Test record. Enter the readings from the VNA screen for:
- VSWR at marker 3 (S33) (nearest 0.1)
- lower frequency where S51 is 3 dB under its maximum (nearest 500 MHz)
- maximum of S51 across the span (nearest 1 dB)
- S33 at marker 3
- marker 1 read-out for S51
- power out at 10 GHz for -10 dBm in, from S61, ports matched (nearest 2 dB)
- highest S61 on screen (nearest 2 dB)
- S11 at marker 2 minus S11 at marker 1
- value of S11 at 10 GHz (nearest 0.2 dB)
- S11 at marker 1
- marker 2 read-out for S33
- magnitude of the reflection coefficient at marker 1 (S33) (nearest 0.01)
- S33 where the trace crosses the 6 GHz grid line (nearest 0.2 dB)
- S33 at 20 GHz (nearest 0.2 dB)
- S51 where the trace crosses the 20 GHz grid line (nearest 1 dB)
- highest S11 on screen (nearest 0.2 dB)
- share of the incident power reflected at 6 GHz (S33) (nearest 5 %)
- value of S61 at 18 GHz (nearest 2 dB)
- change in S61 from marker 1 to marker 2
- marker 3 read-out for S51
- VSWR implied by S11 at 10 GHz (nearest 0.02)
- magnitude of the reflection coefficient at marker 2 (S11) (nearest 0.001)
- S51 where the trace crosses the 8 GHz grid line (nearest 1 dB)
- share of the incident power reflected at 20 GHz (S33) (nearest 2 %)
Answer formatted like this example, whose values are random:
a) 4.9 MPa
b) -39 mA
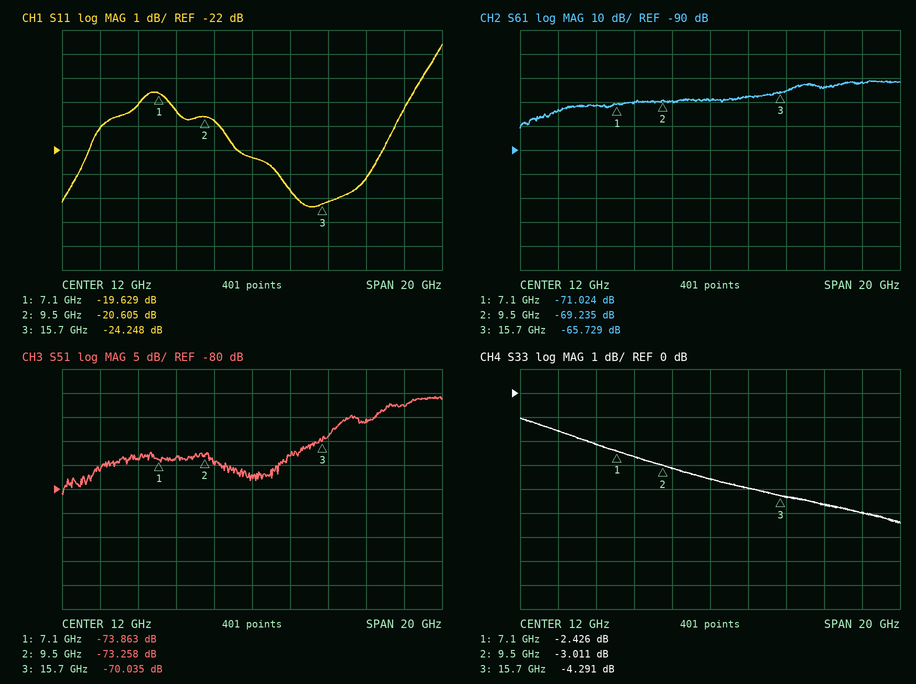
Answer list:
a) 4.1
b) 19.0 GHz
c) -61 dB
d) -4.291 dB
e) -73.863 dB
f) -80 dBm
g) -62 dB
h) -0.976 dB
i) -20.8 dB
j) -19.629 dB
k) -3.011 dB
l) 0.76
m) -2.2 dB
n) -5.0 dB
o) -63 dB
p) -17.6 dB
q) 60 %
r) -64 dB
s) 1.789 dB
t) -70.035 dB
u) 1.20
v) 0.093
w) -73 dB
x) 32 %
